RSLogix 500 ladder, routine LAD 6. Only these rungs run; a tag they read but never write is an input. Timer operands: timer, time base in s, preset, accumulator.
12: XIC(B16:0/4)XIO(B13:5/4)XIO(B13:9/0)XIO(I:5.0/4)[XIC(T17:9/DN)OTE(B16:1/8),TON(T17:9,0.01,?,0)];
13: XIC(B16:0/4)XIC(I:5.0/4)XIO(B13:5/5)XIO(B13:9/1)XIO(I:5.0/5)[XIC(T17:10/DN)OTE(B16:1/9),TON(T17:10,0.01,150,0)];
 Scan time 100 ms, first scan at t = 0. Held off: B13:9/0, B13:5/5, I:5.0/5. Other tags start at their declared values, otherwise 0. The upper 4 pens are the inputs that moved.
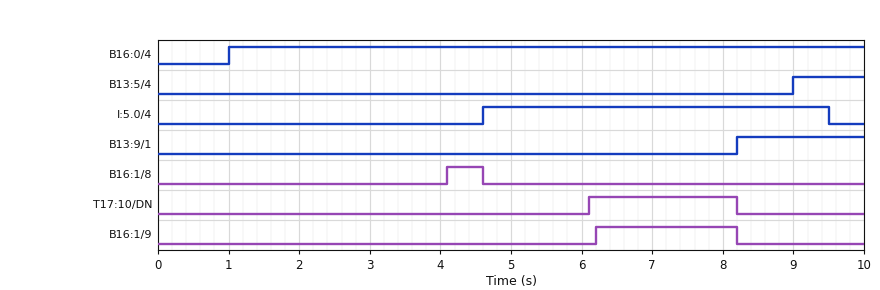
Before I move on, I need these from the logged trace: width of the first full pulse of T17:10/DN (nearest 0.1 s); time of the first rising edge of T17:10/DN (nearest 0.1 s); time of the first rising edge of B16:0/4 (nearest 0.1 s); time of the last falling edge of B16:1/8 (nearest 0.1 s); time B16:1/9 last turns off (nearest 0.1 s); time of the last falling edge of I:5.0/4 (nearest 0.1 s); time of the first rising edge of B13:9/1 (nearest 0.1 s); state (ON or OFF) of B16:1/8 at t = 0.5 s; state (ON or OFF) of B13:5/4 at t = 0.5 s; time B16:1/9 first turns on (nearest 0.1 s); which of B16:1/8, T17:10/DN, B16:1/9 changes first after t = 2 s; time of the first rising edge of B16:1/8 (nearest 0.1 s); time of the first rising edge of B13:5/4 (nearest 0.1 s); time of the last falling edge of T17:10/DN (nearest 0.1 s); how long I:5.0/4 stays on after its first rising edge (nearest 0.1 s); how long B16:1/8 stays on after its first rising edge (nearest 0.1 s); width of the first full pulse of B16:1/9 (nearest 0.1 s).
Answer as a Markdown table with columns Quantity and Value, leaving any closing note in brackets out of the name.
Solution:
| Quantity | Value |
|---|---|
| width of the first full pulse of T17:10/DN | 2.1 s |
| time of the first rising edge of T17:10/DN | 6.1 s |
| time of the first rising edge of B16:0/4 | 1.0 s |
| time of the last falling edge of B16:1/8 | 4.6 s |
| time B16:1/9 last turns off | 8.2 s |
| time of the last falling edge of I:5.0/4 | 9.5 s |
| time of the first rising edge of B13:9/1 | 8.2 s |
| state (ON or OFF) of B16:1/8 at t = 0.5 s | OFF |
| state (ON or OFF) of B13:5/4 at t = 0.5 s | OFF |
| time B16:1/9 first turns on | 6.2 s |
| which of B16:1/8, T17:10/DN, B16:1/9 changes first after t = 2 s | B16:1/8 |
| time of the first rising edge of B16:1/8 | 4.1 s |
| time of the first rising edge of B13:5/4 | 9.0 s |
| time of the last falling edge of T17:10/DN | 8.2 s |
| how long I:5.0/4 stays on after its first rising edge | 4.9 s |
| how long B16:1/8 stays on after its first rising edge | 0.5 s |
| width of the first full pulse of B16:1/9 | 2.0 s |
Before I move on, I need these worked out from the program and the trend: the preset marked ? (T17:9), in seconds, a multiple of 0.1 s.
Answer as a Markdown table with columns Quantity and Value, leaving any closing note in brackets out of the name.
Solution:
| Quantity | Value |
|---|---|
| the preset marked ? (T17:9), in seconds, a multiple of 0.1 s | 3.0 s |
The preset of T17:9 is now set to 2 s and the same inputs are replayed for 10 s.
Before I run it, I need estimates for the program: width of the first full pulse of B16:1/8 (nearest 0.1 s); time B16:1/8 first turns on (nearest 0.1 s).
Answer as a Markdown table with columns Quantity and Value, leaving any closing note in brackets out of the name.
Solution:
| Quantity | Value |
|---|---|
| width of the first full pulse of B16:1/8 | 1.5 s |
| time B16:1/8 first turns on | 3.1 s |
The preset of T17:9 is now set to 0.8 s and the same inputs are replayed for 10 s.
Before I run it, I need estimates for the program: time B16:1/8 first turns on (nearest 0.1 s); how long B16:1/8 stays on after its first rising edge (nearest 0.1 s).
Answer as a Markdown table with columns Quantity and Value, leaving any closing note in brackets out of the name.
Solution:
| Quantity | Value |
|---|---|
| time B16:1/8 first turns on | 1.9 s |
| how long B16:1/8 stays on after its first rising edge | 2.7 s |
